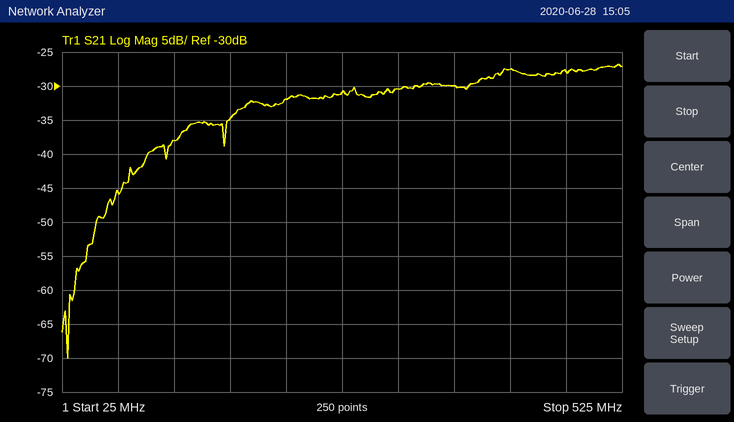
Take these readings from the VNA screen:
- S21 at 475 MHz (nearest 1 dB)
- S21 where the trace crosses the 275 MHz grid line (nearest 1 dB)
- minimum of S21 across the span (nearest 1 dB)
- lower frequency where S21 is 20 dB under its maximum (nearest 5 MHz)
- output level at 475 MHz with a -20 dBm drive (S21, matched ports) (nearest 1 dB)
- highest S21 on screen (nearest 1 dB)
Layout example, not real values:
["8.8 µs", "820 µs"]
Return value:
["-28 dB", "-31 dB", "-70 dB", "70 MHz", "-48 dBm", "-27 dB"]
